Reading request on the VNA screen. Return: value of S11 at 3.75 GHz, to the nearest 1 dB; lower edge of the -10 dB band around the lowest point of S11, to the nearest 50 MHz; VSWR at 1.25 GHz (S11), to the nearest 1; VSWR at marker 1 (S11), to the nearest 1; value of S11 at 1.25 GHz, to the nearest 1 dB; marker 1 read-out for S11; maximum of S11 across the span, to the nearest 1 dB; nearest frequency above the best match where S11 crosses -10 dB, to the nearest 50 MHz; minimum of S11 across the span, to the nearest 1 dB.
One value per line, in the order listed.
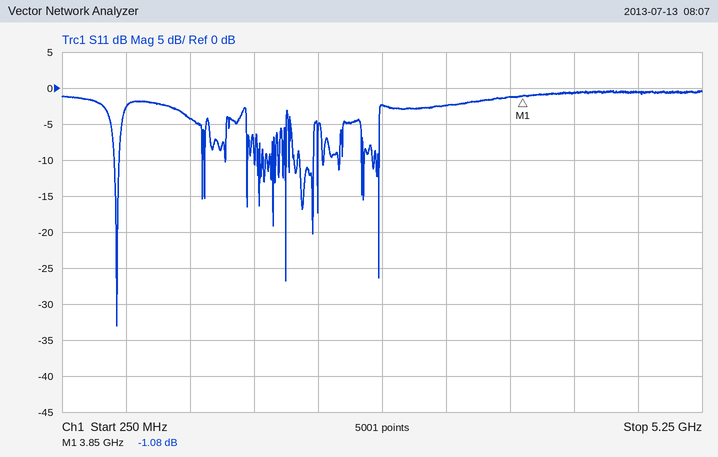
-1 dB
650 MHz
4
16
-4 dB
-1.08 dB
0 dB
700 MHz
-33 dB
